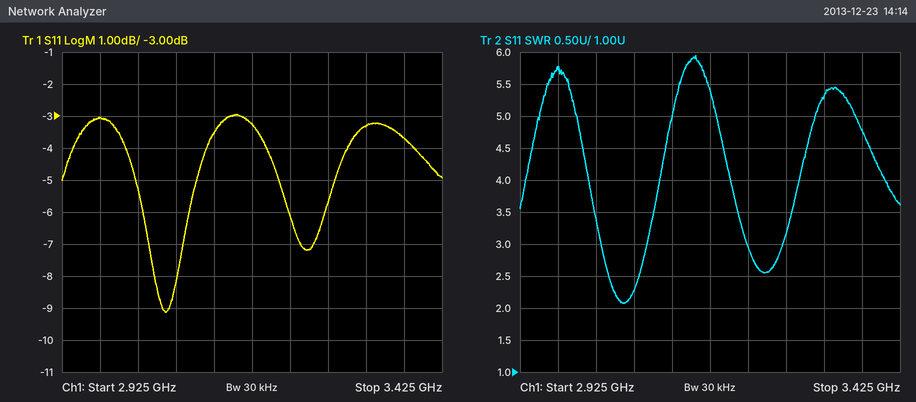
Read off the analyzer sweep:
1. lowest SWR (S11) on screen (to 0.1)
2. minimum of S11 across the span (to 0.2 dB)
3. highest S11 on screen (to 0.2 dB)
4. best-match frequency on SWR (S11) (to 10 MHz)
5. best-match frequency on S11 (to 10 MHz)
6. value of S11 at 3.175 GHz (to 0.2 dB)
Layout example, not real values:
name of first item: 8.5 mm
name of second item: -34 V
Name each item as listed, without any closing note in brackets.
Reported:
lowest SWR (S11) on screen: 2.1
minimum of S11 across the span: -9.2 dB
highest S11 on screen: -3.0 dB
best-match frequency on SWR (S11): 3.06 GHz
best-match frequency on S11: 3.06 GHz
value of S11 at 3.175 GHz: -3.2 dB
